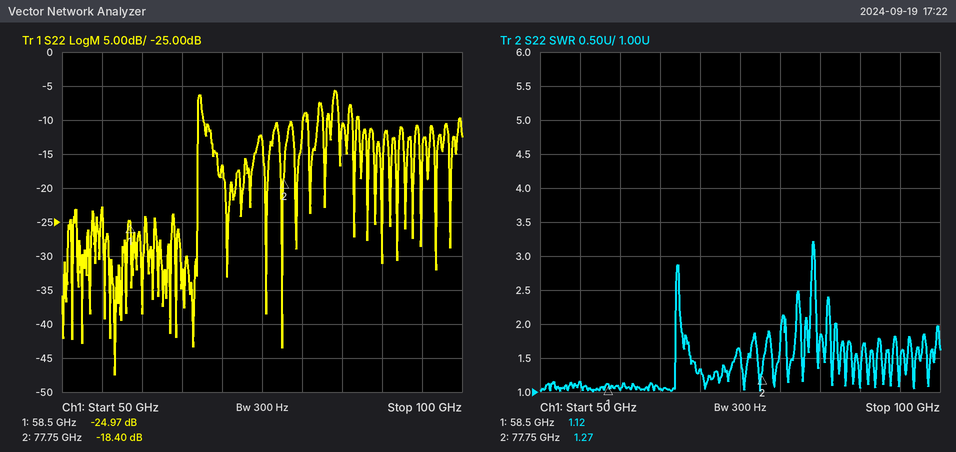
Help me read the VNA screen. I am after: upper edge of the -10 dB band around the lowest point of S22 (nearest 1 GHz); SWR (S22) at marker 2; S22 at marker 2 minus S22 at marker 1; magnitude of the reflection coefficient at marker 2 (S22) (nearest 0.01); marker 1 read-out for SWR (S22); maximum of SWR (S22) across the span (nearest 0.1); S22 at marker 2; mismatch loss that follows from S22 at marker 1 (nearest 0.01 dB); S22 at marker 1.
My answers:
67 GHz
1.27
6.57 dB
0.12
1.12
3.2
-18.40 dB
0.01 dB
-24.97 dB
